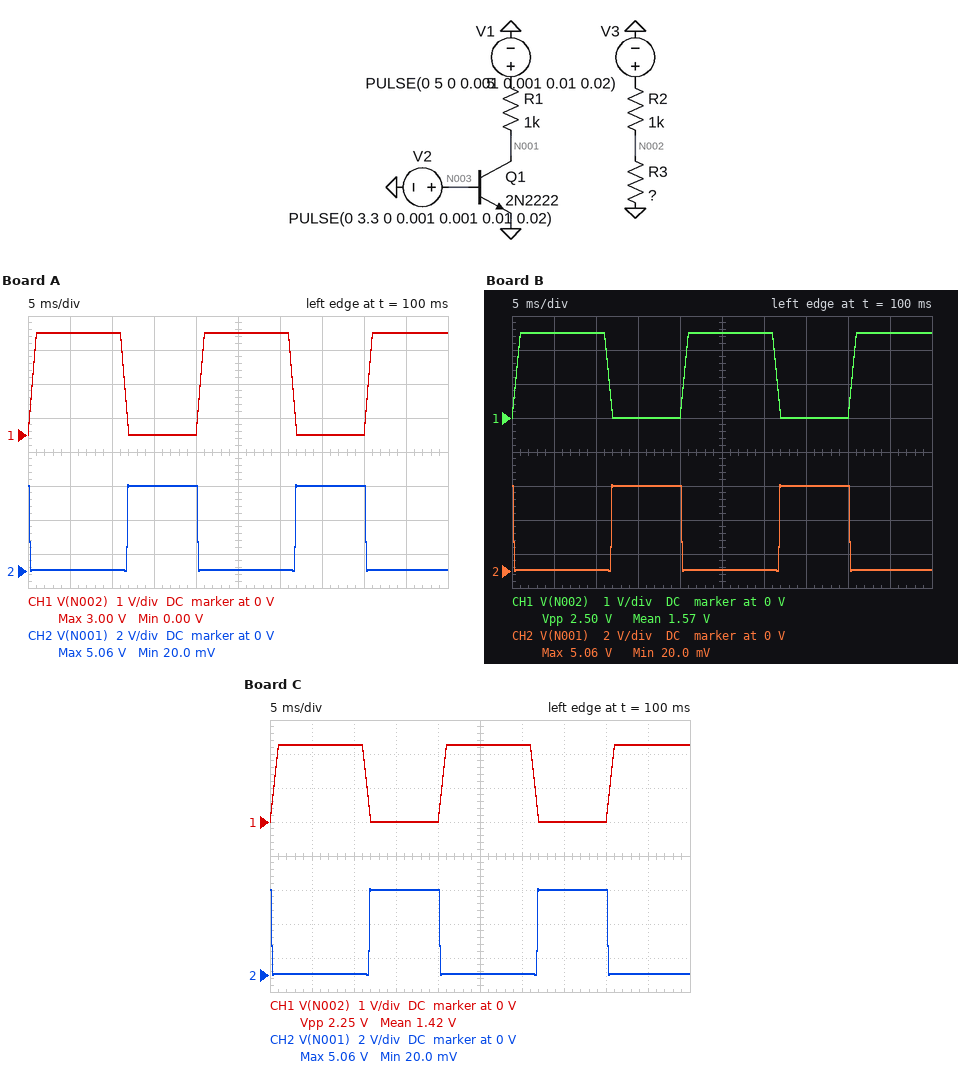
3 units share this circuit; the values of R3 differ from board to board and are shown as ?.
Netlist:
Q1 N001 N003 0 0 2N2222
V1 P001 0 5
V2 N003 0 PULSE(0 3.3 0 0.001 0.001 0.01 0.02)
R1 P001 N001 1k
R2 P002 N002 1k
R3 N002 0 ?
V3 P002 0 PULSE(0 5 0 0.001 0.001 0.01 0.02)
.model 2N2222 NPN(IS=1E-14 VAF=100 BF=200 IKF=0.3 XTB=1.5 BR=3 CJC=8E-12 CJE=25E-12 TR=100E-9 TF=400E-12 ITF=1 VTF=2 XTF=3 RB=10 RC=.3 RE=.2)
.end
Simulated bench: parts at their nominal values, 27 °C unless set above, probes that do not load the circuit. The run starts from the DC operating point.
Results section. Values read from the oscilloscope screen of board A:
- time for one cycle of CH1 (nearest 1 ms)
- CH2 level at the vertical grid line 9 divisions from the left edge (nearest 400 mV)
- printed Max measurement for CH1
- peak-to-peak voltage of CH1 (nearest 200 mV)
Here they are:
20 ms
0 V
3.00 V
3.0 V
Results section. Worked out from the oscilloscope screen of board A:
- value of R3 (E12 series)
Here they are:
1.5 kΩ
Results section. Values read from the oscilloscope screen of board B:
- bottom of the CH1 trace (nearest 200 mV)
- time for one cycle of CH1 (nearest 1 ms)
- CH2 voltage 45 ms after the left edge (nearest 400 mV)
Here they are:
0 V
20 ms
0 V
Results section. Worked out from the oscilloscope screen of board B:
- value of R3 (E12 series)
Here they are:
1 kΩ
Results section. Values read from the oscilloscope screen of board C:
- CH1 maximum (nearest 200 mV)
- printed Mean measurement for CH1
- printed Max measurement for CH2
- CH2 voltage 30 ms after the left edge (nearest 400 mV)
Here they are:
2.2 V
1.42 V
5.06 V
0 V
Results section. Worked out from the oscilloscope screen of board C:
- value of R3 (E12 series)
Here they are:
820 Ω
